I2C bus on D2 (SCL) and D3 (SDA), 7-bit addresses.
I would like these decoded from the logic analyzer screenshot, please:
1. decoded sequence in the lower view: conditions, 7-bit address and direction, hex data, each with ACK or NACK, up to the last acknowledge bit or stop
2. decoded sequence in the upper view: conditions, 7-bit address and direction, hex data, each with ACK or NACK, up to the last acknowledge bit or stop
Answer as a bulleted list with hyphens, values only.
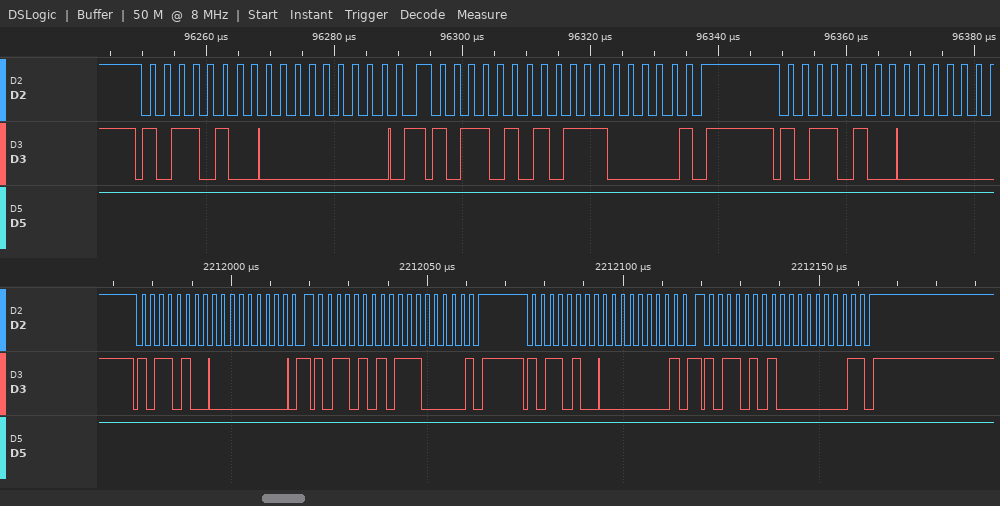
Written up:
- start, address 5A write ACK, 00 ACK, repeated start, address 5A read ACK, E0 NACK, stop, start, address 5A write ACK, 01 ACK, repeated start, address 5A read ACK, 01 NACK, stop
- start, address 5A write ACK, 00 ACK, repeated start, address 5A read ACK, E0 NACK, stop, start, address 5A write ACK
